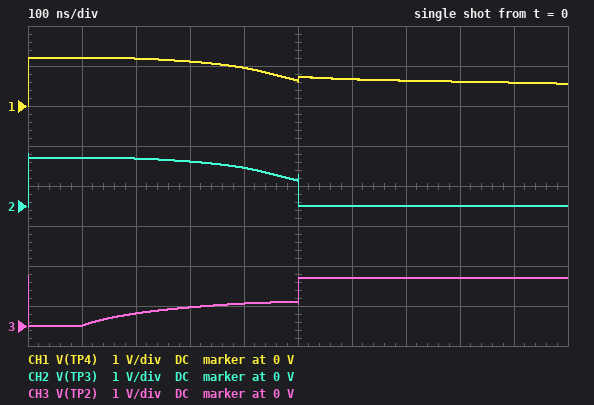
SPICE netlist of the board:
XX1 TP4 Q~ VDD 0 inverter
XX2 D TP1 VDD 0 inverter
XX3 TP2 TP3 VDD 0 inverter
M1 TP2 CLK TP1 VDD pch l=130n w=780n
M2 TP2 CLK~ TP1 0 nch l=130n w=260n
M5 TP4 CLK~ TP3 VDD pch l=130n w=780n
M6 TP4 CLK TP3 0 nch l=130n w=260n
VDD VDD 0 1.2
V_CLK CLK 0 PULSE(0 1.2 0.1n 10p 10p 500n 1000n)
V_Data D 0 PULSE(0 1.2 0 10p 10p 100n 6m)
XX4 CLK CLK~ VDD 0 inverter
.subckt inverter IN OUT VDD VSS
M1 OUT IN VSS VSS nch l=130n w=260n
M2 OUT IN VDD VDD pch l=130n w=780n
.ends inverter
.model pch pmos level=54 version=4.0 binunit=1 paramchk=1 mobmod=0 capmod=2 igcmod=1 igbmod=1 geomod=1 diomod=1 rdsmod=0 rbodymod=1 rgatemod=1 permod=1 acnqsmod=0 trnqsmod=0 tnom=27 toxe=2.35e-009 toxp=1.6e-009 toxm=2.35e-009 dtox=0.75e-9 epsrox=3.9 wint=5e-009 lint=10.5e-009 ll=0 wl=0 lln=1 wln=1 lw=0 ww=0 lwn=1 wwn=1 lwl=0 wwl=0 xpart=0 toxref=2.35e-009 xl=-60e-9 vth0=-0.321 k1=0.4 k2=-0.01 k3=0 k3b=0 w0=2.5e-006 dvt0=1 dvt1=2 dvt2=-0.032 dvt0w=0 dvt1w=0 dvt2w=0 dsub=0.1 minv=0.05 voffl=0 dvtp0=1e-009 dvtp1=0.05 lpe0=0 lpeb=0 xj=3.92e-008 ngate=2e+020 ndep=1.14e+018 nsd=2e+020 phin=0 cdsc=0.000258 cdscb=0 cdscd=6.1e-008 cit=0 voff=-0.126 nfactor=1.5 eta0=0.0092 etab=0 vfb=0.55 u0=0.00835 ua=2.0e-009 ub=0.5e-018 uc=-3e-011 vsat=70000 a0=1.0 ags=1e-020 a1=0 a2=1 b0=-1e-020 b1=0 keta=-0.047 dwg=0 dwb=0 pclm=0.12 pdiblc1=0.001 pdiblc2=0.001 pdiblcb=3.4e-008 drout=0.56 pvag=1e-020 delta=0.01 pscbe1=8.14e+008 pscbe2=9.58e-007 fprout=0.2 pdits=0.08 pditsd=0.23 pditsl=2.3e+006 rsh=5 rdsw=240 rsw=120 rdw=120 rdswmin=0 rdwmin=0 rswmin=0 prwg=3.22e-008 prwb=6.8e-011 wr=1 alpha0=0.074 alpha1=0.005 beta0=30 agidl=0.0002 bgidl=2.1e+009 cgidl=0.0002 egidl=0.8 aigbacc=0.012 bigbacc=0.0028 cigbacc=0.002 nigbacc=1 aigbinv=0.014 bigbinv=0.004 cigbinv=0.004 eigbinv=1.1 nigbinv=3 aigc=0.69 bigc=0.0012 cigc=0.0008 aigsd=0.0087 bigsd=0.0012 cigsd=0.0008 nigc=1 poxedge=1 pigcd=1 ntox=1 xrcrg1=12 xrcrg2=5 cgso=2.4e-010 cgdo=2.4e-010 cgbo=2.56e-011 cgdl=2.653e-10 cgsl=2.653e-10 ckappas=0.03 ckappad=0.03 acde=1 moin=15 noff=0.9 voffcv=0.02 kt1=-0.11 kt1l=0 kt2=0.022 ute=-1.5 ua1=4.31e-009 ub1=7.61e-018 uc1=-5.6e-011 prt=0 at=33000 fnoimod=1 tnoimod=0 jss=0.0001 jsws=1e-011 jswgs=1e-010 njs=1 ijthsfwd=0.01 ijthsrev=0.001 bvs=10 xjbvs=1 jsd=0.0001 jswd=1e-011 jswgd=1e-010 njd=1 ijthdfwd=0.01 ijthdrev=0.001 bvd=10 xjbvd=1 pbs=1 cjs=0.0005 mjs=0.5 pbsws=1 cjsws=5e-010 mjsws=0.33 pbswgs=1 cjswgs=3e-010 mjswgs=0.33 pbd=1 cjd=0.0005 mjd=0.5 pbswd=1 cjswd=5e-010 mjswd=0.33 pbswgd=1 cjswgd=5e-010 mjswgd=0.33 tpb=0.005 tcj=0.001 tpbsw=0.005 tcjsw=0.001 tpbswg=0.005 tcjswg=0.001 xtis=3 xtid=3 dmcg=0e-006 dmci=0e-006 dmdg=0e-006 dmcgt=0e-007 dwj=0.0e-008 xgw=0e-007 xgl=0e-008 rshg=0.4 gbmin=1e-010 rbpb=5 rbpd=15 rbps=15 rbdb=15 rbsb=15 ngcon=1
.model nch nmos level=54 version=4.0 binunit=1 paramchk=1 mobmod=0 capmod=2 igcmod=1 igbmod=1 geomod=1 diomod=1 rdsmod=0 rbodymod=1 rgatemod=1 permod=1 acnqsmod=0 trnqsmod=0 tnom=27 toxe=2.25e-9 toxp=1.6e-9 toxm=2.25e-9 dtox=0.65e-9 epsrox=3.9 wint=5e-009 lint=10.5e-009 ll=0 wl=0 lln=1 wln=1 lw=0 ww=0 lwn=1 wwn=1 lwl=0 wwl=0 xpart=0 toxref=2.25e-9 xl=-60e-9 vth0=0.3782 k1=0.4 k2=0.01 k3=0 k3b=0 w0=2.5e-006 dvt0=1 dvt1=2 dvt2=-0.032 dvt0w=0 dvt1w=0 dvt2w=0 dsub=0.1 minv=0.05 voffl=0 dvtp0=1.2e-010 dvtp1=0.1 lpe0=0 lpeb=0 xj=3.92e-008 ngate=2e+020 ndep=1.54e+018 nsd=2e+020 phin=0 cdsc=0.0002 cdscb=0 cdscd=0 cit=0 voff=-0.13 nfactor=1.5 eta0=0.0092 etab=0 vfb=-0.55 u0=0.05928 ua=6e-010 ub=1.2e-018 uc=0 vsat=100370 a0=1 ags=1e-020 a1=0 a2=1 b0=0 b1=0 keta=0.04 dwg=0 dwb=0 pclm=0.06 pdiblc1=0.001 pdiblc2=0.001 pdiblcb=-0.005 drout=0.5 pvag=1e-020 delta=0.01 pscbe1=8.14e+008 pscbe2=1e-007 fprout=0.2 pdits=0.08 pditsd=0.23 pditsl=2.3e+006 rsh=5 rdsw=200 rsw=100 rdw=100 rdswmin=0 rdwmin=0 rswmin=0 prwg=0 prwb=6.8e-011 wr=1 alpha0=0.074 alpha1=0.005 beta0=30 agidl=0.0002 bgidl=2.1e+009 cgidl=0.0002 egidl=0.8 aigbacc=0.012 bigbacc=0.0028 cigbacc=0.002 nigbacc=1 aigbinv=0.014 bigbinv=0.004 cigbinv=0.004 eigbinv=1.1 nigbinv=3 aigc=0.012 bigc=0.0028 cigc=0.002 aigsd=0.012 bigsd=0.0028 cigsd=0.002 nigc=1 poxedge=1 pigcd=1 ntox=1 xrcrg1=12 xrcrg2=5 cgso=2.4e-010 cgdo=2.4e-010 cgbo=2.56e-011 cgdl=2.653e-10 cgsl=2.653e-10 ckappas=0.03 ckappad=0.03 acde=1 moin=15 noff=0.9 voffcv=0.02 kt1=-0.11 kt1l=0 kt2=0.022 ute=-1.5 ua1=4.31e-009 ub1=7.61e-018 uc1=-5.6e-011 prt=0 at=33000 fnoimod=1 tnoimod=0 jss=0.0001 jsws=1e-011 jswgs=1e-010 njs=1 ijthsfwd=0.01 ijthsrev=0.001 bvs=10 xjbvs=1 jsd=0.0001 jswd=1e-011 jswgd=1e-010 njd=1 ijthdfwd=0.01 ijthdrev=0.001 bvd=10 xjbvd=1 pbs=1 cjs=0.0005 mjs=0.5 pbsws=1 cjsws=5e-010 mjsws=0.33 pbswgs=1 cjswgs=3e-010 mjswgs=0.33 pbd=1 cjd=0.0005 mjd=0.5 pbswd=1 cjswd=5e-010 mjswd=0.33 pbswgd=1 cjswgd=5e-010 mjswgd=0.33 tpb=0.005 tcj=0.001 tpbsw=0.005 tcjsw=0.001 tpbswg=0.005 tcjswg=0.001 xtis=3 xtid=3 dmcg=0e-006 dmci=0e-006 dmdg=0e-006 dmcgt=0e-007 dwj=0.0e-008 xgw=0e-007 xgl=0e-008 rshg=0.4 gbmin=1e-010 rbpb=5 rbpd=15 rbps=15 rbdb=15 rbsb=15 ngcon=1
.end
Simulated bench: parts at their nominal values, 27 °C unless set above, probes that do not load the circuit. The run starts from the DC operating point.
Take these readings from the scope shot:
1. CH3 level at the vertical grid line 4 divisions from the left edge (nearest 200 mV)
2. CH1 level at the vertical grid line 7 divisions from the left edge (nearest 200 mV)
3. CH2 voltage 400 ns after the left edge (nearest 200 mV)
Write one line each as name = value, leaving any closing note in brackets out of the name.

CH3 level at the vertical grid line 4 divisions from the left edge = 600 mV
CH1 level at the vertical grid line 7 divisions from the left edge = 600 mV
CH2 voltage 400 ns after the left edge = 1.0 V
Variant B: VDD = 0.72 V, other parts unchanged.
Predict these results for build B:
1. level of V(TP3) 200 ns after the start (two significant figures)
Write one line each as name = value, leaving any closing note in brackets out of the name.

level of V(TP3) 200 ns after the start = 720 mV
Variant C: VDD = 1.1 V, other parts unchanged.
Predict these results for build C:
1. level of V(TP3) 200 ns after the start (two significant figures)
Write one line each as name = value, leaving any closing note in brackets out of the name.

level of V(TP3) 200 ns after the start = 1.1 V
